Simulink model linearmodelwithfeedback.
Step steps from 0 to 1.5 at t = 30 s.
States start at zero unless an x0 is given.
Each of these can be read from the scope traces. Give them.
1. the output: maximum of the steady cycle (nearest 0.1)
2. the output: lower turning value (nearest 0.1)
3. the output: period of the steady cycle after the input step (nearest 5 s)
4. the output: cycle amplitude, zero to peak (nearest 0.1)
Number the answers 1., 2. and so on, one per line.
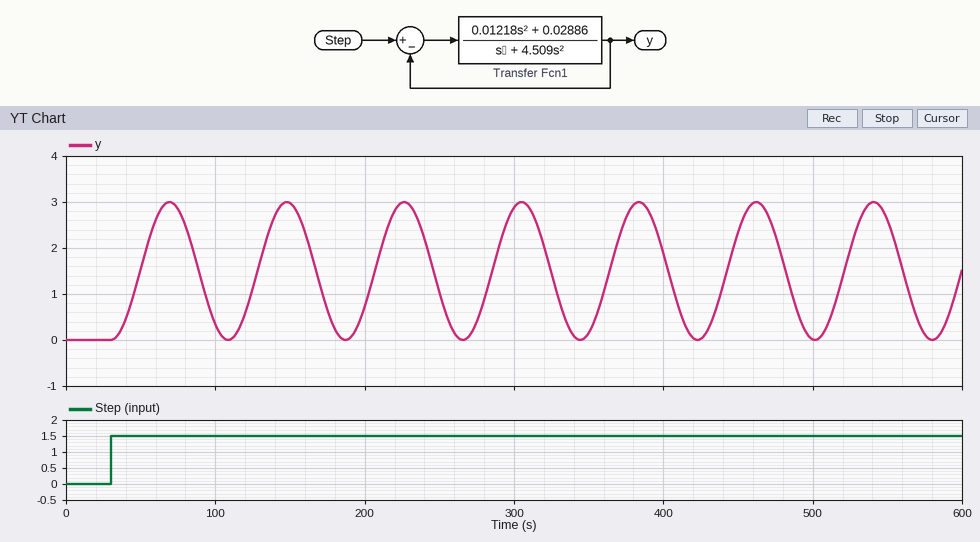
1. 3.0
2. 0.0
3. 80 s
4. 1.5
